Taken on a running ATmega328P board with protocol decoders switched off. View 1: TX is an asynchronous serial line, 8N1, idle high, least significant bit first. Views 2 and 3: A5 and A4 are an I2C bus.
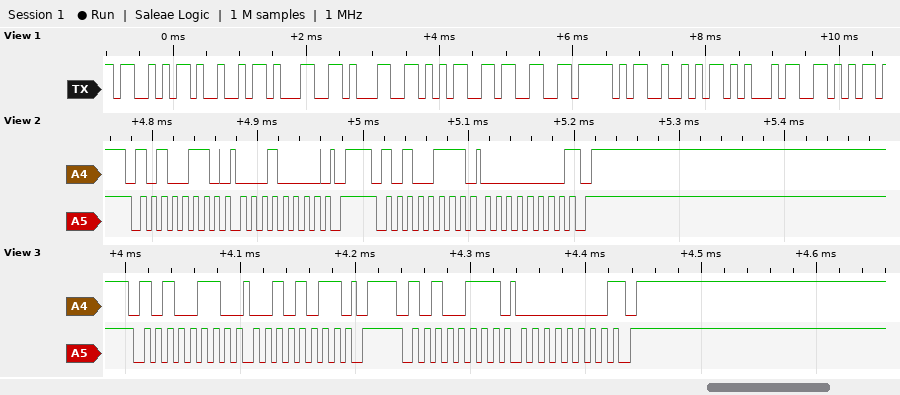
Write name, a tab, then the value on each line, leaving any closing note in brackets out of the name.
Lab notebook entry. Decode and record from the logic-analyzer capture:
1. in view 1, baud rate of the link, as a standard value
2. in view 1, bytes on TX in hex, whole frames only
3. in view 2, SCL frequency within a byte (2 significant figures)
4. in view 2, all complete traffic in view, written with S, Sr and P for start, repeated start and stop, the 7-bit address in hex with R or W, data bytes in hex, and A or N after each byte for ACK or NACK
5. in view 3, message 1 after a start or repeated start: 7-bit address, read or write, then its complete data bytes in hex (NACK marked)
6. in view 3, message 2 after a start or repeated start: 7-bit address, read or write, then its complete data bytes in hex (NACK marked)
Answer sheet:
in view 1, baud rate of the link, as a standard value	9600 baud
in view 1, bytes on TX in hex, whole frames only	53 49 31 31 35 33 5F 52 45 56
in view 2, SCL frequency within a byte	100 kHz
in view 2, all complete traffic in view, written with S, Sr and P for start, repeated start and stop, the 7-bit address in hex with R or W, data bytes in hex, and A or N after each byte for ACK or NACK	S 53W A 10 A P S 53R A 00 N P
in view 3, message 1 after a start or repeated start: 7-bit address, read or write, then its complete data bytes in hex	0x53 write: 2B
in view 3, message 2 after a start or repeated start: 7-bit address, read or write, then its complete data bytes in hex	0x53 read: 00 NACK
